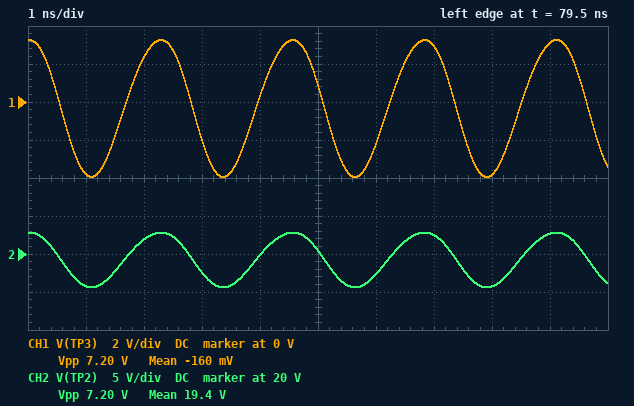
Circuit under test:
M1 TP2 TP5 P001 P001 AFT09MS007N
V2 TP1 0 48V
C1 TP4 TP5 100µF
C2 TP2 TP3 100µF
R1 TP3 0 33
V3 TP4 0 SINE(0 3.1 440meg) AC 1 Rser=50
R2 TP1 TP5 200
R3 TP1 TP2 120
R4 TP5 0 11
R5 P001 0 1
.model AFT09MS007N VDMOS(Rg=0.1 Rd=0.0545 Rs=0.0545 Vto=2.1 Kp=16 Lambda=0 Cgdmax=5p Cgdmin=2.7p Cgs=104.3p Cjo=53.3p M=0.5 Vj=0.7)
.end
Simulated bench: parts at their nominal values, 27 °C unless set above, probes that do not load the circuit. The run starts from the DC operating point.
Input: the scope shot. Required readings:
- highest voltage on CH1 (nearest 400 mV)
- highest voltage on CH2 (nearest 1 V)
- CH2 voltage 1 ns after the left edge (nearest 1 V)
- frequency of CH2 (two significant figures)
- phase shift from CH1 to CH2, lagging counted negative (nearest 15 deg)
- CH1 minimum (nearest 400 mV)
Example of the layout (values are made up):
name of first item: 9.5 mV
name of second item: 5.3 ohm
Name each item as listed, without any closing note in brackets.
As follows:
highest voltage on CH1: 3.2 V
highest voltage on CH2: 23 V
CH2 voltage 1 ns after the left edge: 16 V
frequency of CH2: 440 MHz
phase shift from CH1 to CH2, lagging counted negative: 0 deg
CH1 minimum: -4.0 V
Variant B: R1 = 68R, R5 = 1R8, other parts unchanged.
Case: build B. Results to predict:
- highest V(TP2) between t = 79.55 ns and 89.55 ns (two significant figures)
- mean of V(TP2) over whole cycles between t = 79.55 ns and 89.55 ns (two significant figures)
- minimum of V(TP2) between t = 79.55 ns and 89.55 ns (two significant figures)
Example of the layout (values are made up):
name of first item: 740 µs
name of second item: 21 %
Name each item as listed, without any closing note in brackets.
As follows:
highest V(TP2) between t = 79.55 ns and 89.55 ns: 32 V
mean of V(TP2) over whole cycles between t = 79.55 ns and 89.55 ns: 29 V
minimum of V(TP2) between t = 79.55 ns and 89.55 ns: 25 V
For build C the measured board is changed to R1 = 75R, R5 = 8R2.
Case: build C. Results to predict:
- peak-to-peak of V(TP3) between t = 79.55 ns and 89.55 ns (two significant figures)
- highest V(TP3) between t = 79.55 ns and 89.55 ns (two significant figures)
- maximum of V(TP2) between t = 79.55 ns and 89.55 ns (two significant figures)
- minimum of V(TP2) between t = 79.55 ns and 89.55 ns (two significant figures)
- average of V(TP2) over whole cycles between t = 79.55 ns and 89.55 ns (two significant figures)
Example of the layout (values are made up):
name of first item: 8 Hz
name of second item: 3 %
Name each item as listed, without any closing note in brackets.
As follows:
peak-to-peak of V(TP3) between t = 79.55 ns and 89.55 ns: 3.1 V
highest V(TP3) between t = 79.55 ns and 89.55 ns: 1.4 V
maximum of V(TP2) between t = 79.55 ns and 89.55 ns: 44 V
minimum of V(TP2) between t = 79.55 ns and 89.55 ns: 41 V
average of V(TP2) over whole cycles between t = 79.55 ns and 89.55 ns: 42 V
